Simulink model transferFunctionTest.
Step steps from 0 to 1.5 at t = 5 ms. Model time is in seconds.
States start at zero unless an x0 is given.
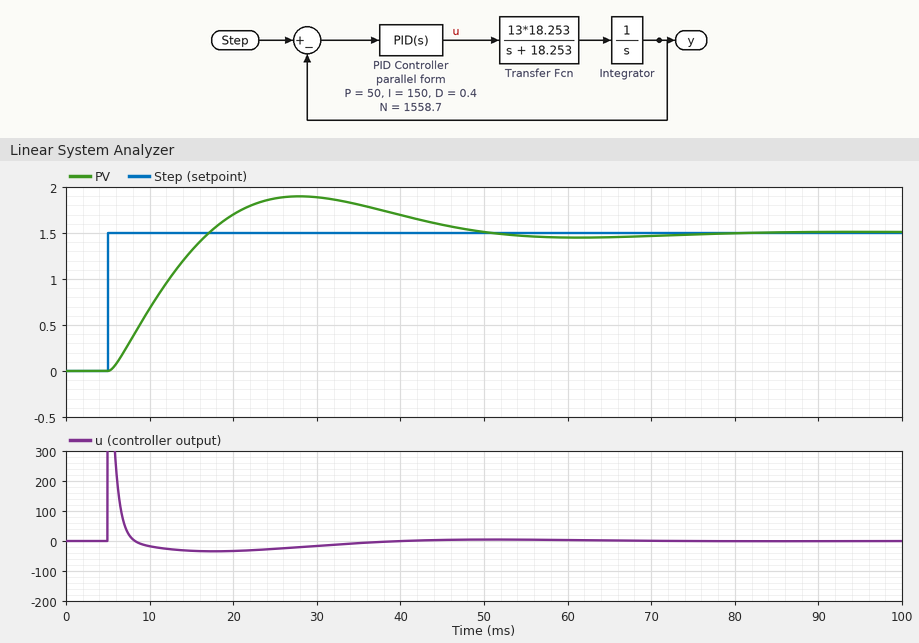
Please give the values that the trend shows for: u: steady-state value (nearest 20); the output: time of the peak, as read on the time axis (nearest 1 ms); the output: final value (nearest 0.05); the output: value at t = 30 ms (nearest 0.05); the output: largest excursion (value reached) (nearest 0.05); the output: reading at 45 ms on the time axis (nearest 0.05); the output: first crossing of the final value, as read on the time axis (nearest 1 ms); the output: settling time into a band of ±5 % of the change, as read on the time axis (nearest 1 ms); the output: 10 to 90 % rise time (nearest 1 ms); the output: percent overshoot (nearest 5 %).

0
28 ms
1.50
1.90
1.90
1.60
17 ms
46 ms
9 ms
25 %
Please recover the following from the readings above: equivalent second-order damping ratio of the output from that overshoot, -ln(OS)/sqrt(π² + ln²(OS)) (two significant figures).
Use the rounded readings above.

0.40
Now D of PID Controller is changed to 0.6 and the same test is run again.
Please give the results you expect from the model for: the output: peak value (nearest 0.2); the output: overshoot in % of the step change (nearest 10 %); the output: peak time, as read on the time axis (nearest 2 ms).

1.8
20 %
26 ms
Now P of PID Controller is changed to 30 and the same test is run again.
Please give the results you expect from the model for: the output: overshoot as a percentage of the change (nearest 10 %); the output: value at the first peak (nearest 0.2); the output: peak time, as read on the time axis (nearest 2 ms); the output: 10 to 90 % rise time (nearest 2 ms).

20 %
1.8
34 ms
12 ms
